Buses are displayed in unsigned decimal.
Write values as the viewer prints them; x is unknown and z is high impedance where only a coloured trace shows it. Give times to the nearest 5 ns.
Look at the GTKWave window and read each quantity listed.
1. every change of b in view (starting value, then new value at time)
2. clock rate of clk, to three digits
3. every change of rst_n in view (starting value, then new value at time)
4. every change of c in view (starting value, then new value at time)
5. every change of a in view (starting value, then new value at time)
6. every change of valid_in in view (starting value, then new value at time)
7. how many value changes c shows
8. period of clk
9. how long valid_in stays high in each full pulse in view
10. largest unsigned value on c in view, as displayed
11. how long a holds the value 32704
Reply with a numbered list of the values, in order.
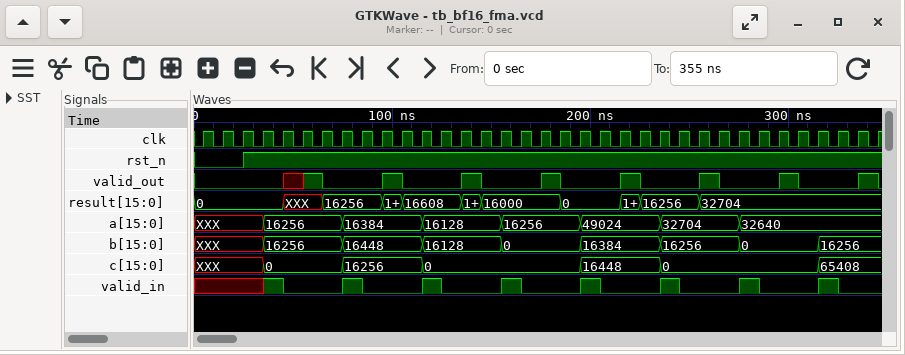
1. XXX, 16256 at 35 ns, 16448 at 75 ns, 16128 at 115 ns, 0 at 155 ns, 16384 at 195 ns, 16256 at 235 ns, 0 at 275 ns, 16256 at 315 ns
2. 100 MHz
3. 0, 1 at 25 ns
4. XXX, 0 at 35 ns, 16256 at 75 ns, 0 at 115 ns, 16448 at 195 ns, 0 at 235 ns, 65408 at 315 ns
5. XXX, 16256 at 35 ns, 16384 at 75 ns, 16128 at 115 ns, 16256 at 155 ns, 49024 at 195 ns, 32704 at 235 ns, 32640 at 275 ns
6. x, 1 at 35 ns, 0 at 45 ns, 1 at 75 ns, 0 at 85 ns, 1 at 115 ns, 0 at 125 ns, 1 at 155 ns, 0 at 165 ns, 1 at 195 ns, 0 at 205 ns, 1 at 235 ns, 0 at 245 ns, 1 at 275 ns, 0 at 285 ns, 1 at 315 ns, 0 at 325 ns
7. 6
8. 10 ns
9. 10 ns, 10 ns, 10 ns, 10 ns, 10 ns, 10 ns, 10 ns
10. 65408
11. 40 ns
